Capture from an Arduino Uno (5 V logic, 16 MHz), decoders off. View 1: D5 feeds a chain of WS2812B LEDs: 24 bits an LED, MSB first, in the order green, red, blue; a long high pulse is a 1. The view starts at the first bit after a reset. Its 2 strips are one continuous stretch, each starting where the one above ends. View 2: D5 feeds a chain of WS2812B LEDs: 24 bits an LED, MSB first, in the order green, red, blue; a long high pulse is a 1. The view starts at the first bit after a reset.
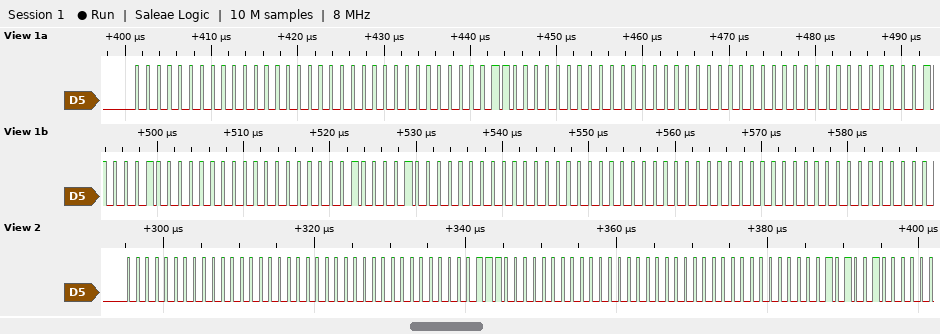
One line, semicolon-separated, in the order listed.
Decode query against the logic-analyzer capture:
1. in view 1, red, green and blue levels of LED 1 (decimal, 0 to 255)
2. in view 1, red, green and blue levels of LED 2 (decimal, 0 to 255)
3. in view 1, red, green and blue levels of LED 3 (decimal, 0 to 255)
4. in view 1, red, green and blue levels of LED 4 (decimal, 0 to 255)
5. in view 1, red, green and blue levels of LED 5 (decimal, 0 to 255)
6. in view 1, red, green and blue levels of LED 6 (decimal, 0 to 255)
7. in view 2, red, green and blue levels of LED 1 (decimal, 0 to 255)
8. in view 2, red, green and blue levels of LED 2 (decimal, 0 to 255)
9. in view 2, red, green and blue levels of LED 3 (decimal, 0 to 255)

0, 0, 0; 96, 0, 0; 0, 0, 0; 0, 66, 0; 0, 66, 0; 0, 0, 0; 0, 0, 0; 7, 0, 0; 0, 0, 0
